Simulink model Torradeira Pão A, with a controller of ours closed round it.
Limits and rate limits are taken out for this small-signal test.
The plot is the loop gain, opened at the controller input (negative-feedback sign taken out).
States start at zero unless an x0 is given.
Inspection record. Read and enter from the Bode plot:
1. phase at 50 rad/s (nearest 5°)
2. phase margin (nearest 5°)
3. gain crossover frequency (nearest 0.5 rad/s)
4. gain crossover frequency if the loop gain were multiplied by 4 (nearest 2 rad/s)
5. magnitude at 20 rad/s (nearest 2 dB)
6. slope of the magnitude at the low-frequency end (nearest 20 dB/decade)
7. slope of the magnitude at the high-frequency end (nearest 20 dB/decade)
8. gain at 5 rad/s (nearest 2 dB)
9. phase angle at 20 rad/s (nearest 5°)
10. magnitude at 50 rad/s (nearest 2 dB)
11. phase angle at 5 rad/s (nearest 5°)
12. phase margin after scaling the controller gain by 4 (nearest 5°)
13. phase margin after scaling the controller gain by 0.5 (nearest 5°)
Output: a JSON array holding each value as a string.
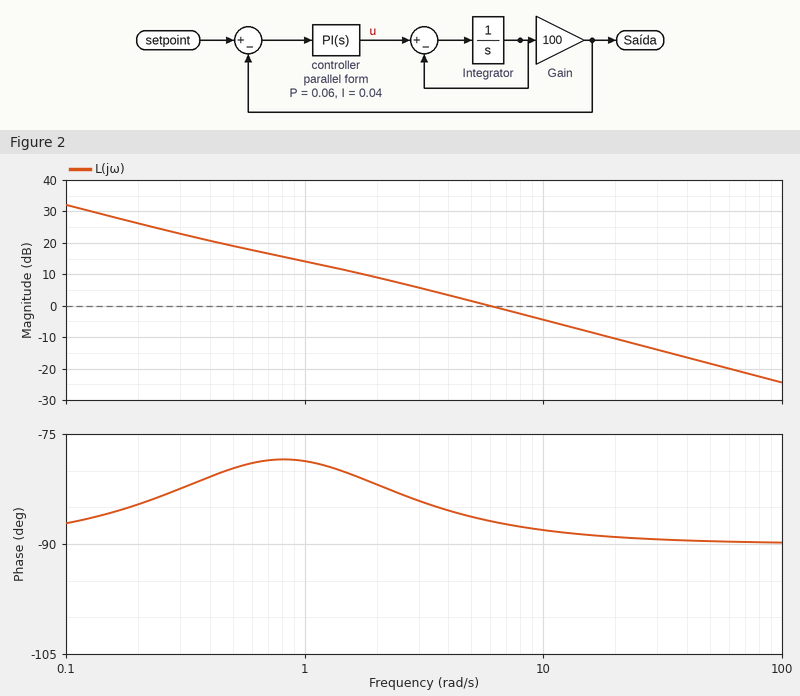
["-90°", "95°", "6.0 rad/s", "24 rad/s", "-10 dB", "-20 dB/decade", "-20 dB/decade", "2 dB", "-90°", "-18 dB", "-85°", "90°", "95°"]
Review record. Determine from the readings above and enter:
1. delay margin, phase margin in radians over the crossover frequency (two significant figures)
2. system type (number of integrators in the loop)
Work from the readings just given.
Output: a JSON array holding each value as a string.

["0.28 s", "1"]
